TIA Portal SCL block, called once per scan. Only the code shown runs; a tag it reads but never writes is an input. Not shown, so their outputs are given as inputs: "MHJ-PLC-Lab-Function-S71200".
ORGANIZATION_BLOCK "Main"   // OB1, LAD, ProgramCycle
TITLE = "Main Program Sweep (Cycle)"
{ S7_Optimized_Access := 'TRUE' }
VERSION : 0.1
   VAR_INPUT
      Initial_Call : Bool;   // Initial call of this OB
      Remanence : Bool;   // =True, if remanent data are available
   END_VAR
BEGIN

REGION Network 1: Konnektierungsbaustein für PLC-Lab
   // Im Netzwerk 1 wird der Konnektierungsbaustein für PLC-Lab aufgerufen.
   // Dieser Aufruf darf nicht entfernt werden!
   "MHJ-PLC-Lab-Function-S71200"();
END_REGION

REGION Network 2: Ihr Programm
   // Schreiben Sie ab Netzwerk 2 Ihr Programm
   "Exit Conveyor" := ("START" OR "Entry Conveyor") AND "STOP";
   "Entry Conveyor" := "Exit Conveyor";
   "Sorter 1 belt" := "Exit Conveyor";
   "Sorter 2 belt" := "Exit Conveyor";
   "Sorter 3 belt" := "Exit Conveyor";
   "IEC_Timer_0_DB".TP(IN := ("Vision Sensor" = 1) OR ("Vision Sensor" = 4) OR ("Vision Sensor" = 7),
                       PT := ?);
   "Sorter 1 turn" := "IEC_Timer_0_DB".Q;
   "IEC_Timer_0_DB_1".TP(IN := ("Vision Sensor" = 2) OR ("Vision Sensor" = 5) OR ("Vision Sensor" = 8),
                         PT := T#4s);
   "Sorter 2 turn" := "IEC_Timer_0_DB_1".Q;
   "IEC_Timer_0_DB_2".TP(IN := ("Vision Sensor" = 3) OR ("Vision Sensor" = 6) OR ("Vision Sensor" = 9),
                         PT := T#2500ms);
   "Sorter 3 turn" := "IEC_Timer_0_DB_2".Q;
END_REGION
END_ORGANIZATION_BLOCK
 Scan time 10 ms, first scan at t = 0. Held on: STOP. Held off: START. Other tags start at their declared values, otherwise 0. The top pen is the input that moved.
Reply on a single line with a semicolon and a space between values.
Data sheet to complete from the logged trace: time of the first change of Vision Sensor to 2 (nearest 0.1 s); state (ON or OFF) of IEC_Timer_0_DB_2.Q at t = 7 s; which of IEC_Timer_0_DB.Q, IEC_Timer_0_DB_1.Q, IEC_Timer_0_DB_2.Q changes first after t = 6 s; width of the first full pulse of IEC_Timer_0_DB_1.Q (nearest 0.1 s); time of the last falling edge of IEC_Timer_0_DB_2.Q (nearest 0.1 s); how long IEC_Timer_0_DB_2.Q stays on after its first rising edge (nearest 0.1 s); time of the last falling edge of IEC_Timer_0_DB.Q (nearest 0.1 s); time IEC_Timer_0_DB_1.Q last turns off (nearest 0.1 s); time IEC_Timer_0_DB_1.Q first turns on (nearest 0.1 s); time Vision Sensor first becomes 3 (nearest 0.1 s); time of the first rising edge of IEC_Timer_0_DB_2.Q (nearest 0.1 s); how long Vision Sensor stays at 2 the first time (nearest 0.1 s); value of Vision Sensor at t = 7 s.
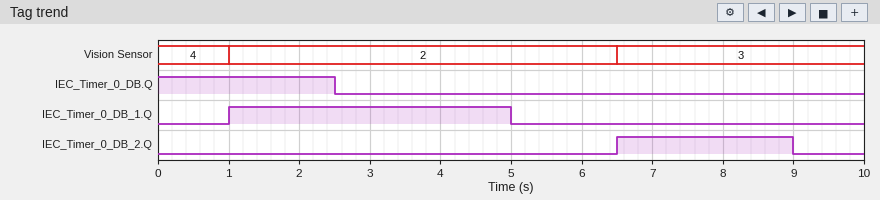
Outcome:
1.0 s; ON; IEC_Timer_0_DB_2.Q; 4.0 s; 9.0 s; 2.5 s; 2.5 s; 5.0 s; 1.0 s; 6.5 s; 6.5 s; 5.5 s; 3
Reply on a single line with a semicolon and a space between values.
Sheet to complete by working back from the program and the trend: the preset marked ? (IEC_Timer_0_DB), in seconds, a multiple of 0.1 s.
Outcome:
2.5 s
